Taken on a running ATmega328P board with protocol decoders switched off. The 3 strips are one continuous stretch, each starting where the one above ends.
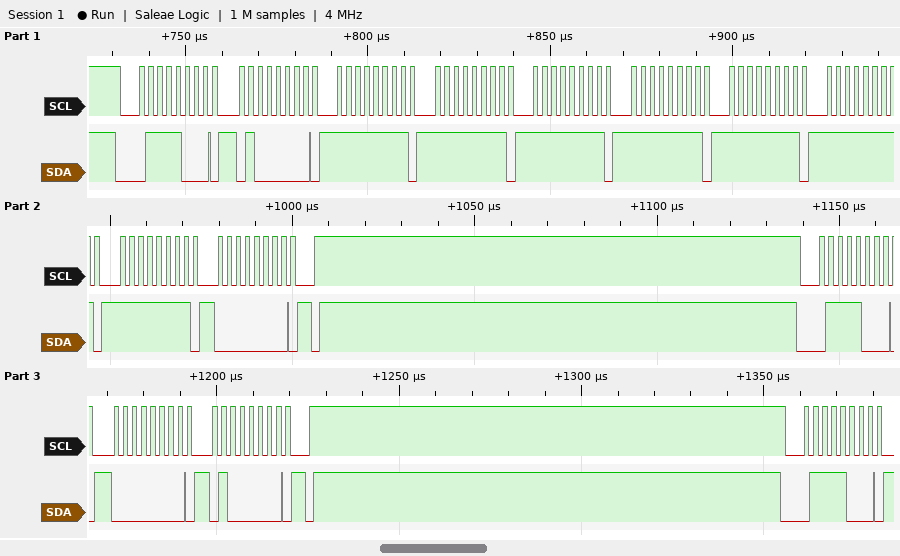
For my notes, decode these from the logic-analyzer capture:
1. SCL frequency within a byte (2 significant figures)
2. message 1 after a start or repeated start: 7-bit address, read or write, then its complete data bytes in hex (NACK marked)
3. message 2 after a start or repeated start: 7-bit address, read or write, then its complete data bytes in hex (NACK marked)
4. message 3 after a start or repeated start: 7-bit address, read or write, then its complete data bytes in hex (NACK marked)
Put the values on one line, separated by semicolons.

400 kHz; 0x3C write: 40 FF FF FF FF FF FF FF 00; 0x3C write: 00 40; 0x3C write
